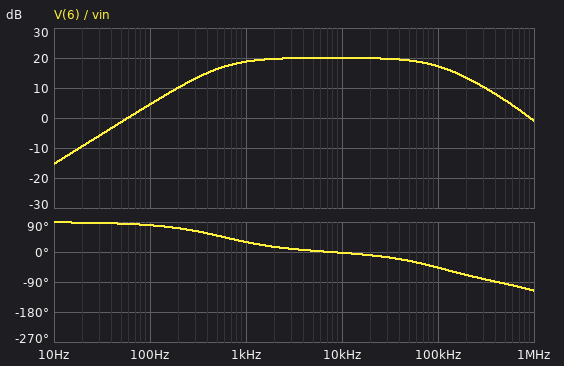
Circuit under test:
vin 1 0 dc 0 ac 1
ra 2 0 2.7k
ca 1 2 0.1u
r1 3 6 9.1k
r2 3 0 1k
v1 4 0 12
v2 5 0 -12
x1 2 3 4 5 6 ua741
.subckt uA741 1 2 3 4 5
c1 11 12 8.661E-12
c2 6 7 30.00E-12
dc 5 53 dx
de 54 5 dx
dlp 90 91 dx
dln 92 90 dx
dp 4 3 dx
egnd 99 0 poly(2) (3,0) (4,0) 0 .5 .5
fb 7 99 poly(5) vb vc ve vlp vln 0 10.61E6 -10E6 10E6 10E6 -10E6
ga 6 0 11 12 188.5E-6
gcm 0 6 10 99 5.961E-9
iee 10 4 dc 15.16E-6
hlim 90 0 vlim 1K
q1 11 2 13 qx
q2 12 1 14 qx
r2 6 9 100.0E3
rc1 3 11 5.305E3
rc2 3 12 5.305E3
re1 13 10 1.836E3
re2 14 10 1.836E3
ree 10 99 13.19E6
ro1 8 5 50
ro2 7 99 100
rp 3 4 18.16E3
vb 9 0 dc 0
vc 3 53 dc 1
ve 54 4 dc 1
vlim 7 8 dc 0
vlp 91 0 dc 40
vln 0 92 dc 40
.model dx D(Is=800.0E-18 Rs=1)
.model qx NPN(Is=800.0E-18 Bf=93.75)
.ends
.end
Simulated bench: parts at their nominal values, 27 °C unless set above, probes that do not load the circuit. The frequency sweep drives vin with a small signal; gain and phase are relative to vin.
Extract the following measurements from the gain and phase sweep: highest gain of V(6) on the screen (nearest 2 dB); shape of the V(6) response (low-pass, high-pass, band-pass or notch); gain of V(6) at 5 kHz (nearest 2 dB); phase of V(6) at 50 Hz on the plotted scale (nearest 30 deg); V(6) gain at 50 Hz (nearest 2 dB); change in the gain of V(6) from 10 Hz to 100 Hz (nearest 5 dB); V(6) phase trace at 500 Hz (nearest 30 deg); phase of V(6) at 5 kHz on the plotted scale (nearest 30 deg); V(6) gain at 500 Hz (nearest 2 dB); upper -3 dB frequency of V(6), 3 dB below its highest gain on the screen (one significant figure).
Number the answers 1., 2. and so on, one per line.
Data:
1. 20 dB
2. band-pass
3. 20 dB
4. 90 deg
5. -2 dB
6. 20 dB
7. 60 deg
8. 0 deg
9. 16 dB
10. 100 kHz
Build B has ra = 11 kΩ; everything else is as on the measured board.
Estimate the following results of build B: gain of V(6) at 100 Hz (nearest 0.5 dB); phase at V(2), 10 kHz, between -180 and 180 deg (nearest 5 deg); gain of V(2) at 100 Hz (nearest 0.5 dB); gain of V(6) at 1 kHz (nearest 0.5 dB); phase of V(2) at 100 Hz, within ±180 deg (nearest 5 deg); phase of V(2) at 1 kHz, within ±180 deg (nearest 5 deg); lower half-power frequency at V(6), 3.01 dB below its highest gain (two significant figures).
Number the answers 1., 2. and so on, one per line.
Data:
1. 15.0 dB
2. 0 deg
3. -5.0 dB
4. 20.0 dB
5. 55 deg
6. 10 deg
7. 140 Hz
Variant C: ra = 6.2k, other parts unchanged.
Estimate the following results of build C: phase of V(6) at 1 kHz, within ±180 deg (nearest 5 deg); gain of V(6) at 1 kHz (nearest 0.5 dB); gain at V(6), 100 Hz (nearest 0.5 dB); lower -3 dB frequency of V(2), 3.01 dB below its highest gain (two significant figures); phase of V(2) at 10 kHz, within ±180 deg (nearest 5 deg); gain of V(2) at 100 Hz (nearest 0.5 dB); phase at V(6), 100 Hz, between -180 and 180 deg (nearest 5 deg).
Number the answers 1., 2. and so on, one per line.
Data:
1. 15 deg
2. 20.0 dB
3. 11.5 dB
4. 260 Hz
5. 0 deg
6. -9.0 dB
7. 70 deg
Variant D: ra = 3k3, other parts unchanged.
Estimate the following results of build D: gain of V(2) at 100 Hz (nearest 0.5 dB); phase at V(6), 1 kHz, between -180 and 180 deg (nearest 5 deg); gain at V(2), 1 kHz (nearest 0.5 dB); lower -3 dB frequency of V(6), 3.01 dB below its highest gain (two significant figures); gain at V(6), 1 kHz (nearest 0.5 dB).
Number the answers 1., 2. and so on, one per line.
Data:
1. -14.0 dB
2. 25 deg
3. -1.0 dB
4. 480 Hz
5. 19.0 dB
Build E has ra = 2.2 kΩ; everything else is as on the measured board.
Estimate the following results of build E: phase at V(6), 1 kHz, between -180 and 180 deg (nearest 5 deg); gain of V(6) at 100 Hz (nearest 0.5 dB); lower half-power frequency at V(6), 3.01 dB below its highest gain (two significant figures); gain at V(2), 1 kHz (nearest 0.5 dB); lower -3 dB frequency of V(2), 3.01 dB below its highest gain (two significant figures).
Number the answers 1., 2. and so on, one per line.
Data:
1. 35 deg
2. 3.0 dB
3. 710 Hz
4. -2.0 dB
5. 720 Hz
